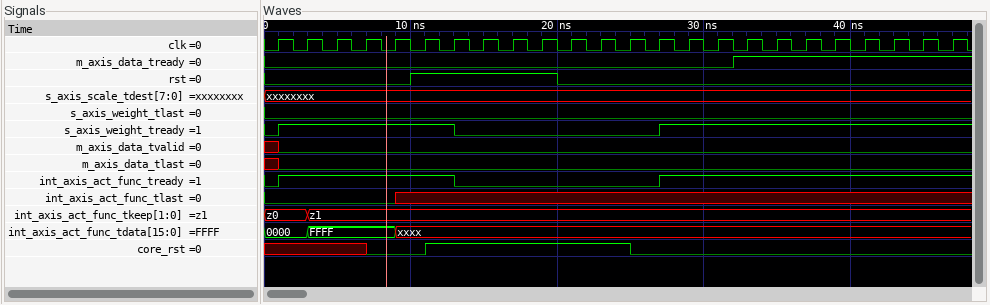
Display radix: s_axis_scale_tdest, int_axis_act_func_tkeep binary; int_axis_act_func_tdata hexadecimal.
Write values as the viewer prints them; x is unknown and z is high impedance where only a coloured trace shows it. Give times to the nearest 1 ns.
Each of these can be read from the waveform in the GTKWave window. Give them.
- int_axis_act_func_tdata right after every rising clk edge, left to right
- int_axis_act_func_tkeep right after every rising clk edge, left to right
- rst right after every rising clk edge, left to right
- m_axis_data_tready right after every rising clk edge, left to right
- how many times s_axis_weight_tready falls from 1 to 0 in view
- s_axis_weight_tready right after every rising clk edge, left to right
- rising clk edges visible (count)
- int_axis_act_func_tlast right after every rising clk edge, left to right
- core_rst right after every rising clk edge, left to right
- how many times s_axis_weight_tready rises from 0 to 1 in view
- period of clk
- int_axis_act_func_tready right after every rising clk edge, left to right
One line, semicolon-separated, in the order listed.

0000, FFFF, FFFF, FFFF, xxxx, xxxx, xxxx, xxxx, xxxx, xxxx, xxxx, xxxx, xxxx, xxxx, xxxx, xxxx, xxxx, xxxx, xxxx, xxxx, xxxx, xxxx, xxxx, xxxx; z0, z1, z1, z1, z1, z1, z1, z1, z1, z1, z1, z1, z1, z1, z1, z1, z1, z1, z1, z1, z1, z1, z1, z1; 0 0 0 0 0 1 1 1 1 1 0 0 0 0 0 0 0 0 0 0 0 0 0 0; 0 0 0 0 0 0 0 0 0 0 0 0 0 0 0 0 1 1 1 1 1 1 1 1; 1; 1 1 1 1 1 1 0 0 0 0 0 0 0 1 1 1 1 1 1 1 1 1 1 1; 24; 0 0 0 0 x x x x x x x x x x x x x x x x x x x x; x x x 0 0 1 1 1 1 1 1 1 0 0 0 0 0 0 0 0 0 0 0 0; 2; 2 ns; 1 1 1 1 1 1 0 0 0 0 0 0 0 1 1 1 1 1 1 1 1 1 1 1
